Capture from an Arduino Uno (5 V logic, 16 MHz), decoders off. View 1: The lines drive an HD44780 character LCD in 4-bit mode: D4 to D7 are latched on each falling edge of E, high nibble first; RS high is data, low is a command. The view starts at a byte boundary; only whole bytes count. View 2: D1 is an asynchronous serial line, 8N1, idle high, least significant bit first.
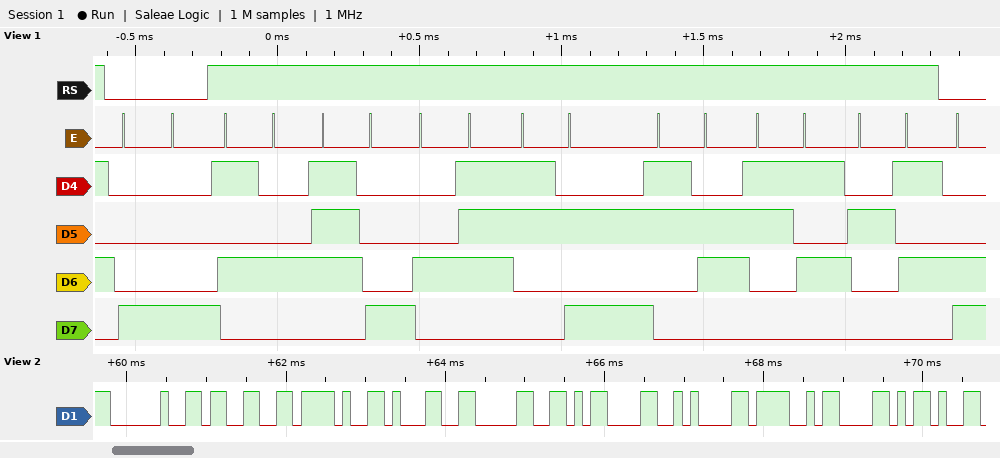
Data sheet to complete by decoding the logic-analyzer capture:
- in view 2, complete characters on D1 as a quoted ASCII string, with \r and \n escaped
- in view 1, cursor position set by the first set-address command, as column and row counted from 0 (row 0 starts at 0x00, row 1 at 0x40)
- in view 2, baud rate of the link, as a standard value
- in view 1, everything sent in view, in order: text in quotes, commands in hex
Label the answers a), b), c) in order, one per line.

a) " 3/10\r\nOX"
b) column 8, row 0
c) 9600 baud
d) 0x88 "TxG:65%"
